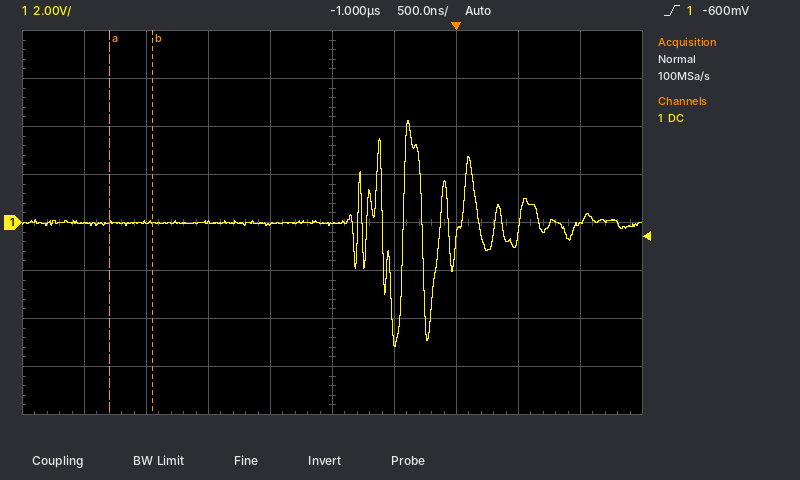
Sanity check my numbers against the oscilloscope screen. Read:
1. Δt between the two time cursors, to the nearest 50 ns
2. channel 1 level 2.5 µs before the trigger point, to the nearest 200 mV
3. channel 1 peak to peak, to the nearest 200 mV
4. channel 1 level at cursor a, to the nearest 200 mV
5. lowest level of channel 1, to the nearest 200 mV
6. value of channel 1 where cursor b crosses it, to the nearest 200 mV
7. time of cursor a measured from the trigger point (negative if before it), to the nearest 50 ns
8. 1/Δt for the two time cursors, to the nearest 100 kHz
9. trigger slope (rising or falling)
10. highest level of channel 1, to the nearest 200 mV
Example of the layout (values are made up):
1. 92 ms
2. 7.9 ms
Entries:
1. 350 ns
2. 0.0 V
3. 9.4 V
4. 0.0 V
5. -5.2 V
6. 0.0 V
7. -2.80 µs
8. 2.9 MHz
9. rising
10. 4.2 V
